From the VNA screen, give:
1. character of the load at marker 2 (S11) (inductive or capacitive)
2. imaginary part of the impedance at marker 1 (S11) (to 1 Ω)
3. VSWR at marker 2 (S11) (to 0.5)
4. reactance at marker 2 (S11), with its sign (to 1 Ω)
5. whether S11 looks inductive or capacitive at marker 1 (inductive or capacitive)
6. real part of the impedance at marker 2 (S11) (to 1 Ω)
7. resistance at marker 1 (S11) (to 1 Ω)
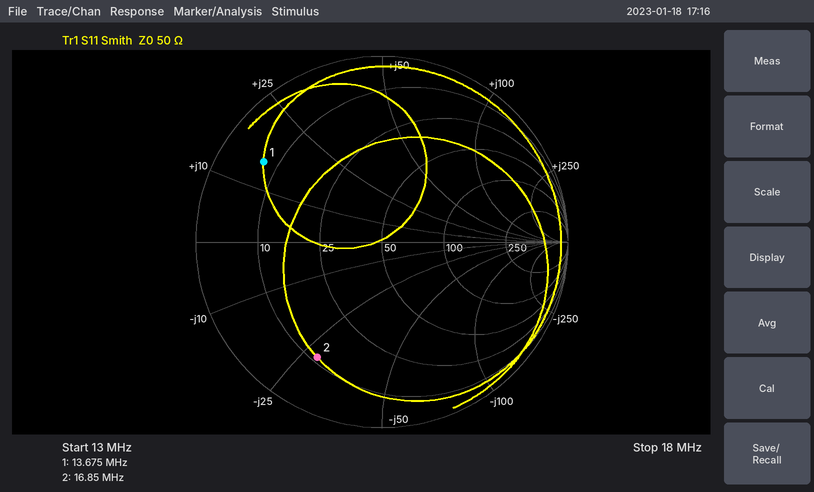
capacitive
+15 Ω
6.0
-28 Ω
inductive
11 Ω
7 Ω
